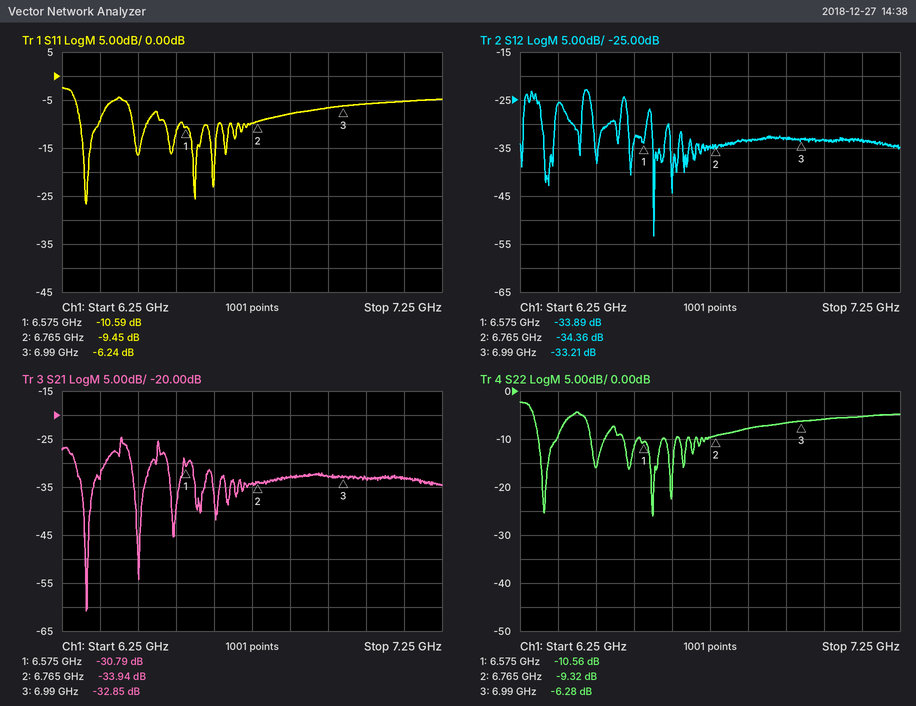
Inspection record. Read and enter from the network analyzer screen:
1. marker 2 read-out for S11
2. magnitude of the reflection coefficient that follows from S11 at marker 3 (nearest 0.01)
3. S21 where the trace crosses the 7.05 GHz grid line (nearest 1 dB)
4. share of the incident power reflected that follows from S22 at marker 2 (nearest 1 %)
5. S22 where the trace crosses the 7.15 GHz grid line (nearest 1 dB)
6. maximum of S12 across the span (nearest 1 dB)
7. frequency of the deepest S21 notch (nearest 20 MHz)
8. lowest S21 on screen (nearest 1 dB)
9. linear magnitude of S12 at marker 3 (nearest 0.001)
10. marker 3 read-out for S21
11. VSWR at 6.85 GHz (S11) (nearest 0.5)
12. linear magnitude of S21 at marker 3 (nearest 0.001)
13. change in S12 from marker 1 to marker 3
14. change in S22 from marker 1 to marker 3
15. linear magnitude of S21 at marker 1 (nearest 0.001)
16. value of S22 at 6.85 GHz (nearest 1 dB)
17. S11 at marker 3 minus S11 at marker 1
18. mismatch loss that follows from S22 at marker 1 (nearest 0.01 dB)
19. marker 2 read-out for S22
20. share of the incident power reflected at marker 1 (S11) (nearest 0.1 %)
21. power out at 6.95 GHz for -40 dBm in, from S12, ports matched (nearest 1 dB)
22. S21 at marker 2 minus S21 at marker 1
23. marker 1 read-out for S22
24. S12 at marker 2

-9.45 dB
0.49
-33 dB
12 %
-5 dB
-23 dB
6.32 GHz
-61 dB
0.022
-32.85 dB
2.5
0.023
0.68 dB
4.28 dB
0.029
-8 dB
4.35 dB
0.40 dB
-9.32 dB
8.7 %
-73 dBm
-3.15 dB
-10.56 dB
-34.36 dB
